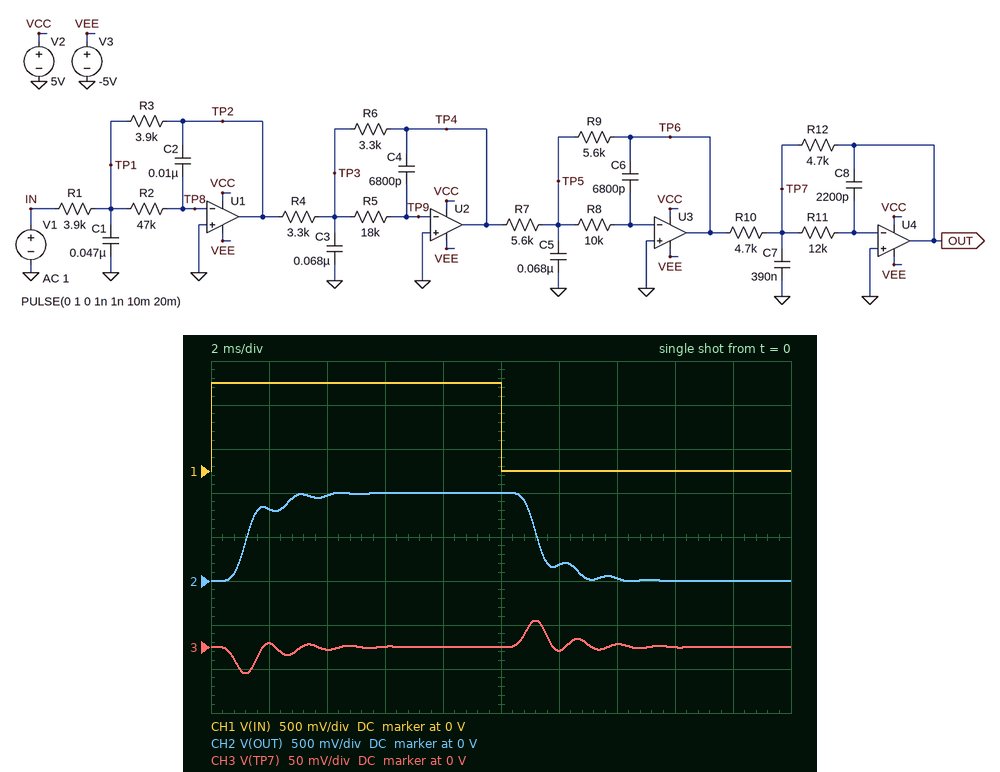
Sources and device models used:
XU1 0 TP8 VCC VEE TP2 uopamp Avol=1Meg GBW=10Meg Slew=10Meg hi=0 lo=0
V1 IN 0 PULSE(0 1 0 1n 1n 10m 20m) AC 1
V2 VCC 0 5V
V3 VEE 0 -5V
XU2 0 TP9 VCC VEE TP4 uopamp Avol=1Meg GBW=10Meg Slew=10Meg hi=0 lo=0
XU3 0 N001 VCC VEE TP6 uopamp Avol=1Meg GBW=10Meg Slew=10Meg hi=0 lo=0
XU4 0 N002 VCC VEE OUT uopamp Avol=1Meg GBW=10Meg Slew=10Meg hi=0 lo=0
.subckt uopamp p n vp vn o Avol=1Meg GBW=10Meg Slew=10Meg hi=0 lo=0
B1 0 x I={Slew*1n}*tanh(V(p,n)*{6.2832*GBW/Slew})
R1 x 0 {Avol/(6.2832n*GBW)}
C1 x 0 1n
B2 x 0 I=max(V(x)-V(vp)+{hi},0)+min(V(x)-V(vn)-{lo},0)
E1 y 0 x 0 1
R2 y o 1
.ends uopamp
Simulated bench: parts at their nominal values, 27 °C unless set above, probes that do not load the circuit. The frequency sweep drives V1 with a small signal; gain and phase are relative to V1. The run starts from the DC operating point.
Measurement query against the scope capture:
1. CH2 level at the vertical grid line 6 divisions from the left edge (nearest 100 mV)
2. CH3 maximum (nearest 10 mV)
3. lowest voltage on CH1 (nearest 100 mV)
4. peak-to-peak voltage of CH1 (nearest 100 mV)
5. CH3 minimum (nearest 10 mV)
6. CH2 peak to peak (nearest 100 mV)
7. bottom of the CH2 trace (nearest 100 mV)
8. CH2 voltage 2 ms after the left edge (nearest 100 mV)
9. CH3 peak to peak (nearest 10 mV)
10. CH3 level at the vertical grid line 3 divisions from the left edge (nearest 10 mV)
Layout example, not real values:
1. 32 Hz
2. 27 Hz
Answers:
1. 200 mV
2. 30 mV
3. 0 V
4. 1.0 V
5. -30 mV
6. 1.0 V
7. 0 V
8. 800 mV
9. 60 mV
10. 0 V
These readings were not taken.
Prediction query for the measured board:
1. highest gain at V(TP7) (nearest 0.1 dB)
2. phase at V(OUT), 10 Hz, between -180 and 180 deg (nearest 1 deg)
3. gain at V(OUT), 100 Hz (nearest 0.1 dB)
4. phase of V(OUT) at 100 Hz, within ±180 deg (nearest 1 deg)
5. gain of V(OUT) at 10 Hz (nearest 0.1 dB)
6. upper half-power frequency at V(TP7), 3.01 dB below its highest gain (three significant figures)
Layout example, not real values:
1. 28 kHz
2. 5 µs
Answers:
1. -21.8 dB
2. -5 deg
3. -1.0 dB
4. -51 deg
5. 0 dB
6. 786 Hz
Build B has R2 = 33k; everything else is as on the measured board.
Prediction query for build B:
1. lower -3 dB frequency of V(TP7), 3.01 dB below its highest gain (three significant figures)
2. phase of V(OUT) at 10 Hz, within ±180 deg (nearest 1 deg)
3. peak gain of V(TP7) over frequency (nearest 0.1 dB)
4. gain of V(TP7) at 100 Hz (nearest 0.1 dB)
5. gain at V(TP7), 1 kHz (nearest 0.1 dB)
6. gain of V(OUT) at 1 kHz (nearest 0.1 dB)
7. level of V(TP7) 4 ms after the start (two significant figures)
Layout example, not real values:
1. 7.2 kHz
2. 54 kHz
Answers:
1. 571 Hz
2. -4 deg
3. -18.8 dB
4. -36.0 dB
5. -34.1 dB
6. -18.5 dB
7. -3.9 mV
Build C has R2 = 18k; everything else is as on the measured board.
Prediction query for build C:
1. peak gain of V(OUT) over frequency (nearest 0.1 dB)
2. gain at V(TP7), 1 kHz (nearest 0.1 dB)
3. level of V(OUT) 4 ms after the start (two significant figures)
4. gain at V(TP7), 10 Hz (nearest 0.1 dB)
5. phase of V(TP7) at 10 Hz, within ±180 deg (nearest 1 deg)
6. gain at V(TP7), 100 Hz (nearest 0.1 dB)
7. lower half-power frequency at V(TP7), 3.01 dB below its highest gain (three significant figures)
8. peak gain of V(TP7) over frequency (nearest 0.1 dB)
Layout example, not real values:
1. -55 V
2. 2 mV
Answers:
1. 4.7 dB
2. -28.9 dB
3. 990 mV
4. -55.6 dB
5. -93 deg
6. -35.6 dB
7. 584 Hz
8. -14.1 dB
